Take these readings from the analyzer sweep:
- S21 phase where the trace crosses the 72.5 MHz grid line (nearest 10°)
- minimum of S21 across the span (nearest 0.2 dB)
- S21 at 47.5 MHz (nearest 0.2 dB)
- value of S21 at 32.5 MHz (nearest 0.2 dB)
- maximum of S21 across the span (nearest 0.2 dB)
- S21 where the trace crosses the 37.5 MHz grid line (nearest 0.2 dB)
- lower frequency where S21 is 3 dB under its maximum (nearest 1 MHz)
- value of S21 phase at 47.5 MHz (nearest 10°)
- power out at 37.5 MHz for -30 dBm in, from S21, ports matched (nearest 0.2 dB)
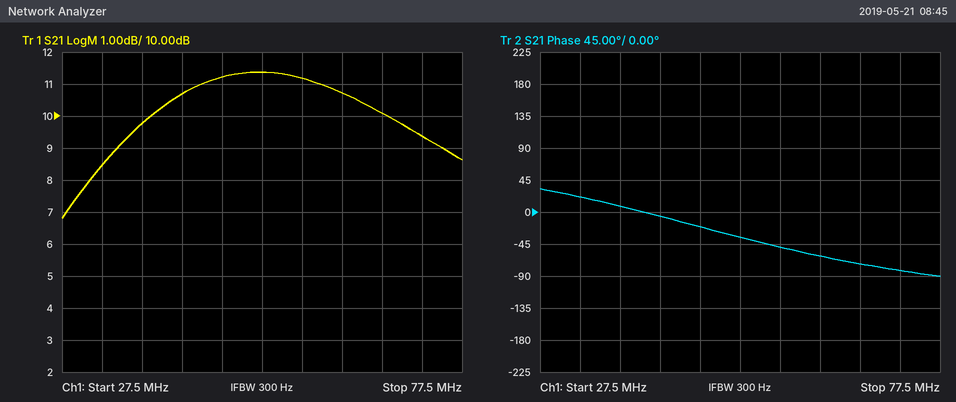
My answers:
-80°
6.8 dB
11.2 dB
8.4 dB
11.4 dB
9.8 dB
32 MHz
-20°
-20.2 dBm
